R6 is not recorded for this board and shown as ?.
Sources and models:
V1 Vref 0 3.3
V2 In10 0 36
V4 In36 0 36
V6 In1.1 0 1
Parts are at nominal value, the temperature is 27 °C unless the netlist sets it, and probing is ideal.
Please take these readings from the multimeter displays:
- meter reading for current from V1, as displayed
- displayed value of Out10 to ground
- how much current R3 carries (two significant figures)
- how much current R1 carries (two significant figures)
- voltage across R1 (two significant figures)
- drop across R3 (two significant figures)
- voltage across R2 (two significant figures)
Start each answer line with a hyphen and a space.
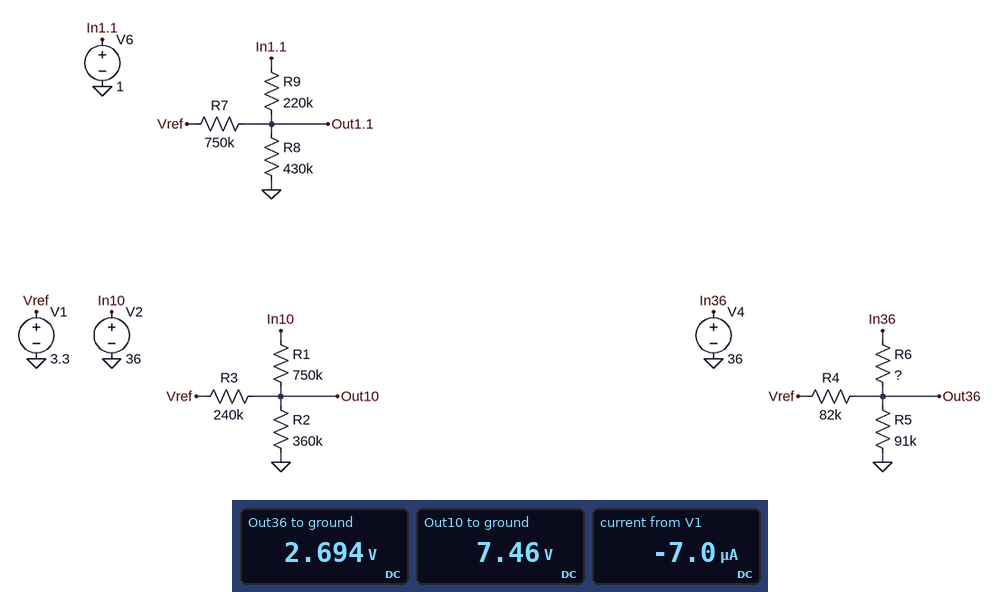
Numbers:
- -7.0 µA
- 7.46 V
- 17 µA
- 38 µA
- 29 V
- 4.2 V
- 7.5 V
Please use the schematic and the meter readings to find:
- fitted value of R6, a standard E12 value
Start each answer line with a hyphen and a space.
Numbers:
- 1.5 MΩ
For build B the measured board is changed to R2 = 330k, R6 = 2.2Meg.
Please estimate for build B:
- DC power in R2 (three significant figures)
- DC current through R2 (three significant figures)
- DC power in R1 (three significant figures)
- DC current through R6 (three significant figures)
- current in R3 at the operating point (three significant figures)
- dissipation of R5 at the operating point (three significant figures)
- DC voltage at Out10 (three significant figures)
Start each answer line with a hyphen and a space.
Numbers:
- 159 µW
- 21.9 µA
- 1.10 mW
- 15.3 µA
- 16.4 µA
- 63.0 µW
- 7.24 V
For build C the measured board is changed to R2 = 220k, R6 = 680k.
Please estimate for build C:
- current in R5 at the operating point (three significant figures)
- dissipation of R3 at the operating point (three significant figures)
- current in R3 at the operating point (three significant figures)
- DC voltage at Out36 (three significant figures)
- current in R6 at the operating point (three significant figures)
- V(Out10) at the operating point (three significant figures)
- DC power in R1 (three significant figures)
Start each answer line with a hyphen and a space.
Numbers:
- 41.5 µA
- 33.8 µW
- 11.9 µA
- 3.78 V
- 47.4 µA
- 6.15 V
- 1.19 mW
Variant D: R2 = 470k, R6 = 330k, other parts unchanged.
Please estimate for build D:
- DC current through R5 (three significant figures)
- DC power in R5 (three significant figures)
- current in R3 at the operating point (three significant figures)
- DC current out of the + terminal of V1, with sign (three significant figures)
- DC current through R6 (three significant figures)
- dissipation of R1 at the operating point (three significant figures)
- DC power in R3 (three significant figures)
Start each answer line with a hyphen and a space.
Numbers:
- 62.6 µA
- 357 µW
- 20.0 µA
- -46.3 µA
- 91.8 µA
- 1.04 mW
- 95.8 µW
